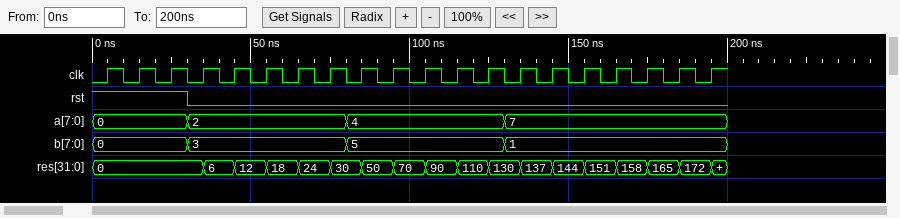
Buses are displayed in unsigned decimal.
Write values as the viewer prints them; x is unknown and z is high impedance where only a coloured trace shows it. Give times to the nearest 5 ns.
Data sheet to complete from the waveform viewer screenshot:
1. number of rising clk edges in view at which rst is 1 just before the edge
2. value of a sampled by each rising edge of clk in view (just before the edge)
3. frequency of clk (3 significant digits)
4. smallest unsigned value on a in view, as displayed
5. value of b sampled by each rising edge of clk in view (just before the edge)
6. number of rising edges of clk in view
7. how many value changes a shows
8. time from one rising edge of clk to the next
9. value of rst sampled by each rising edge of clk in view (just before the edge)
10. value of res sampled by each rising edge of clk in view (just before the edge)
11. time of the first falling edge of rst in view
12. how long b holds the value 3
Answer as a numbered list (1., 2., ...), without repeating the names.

1. 3
2. 0, 0, 0, 2, 2, 2, 2, 2, 4, 4, 4, 4, 4, 7, 7, 7, 7, 7, 7, 7
3. 100 MHz
4. 0
5. 0, 0, 0, 3, 3, 3, 3, 3, 5, 5, 5, 5, 5, 1, 1, 1, 1, 1, 1, 1
6. 20
7. 3
8. 10 ns
9. 1 1 1 0 0 0 0 0 0 0 0 0 0 0 0 0 0 0 0 0
10. 0, 0, 0, 0, 6, 12, 18, 24, 30, 50, 70, 90, 110, 130, 137, 144, 151, 158, 165, 172
11. 30 ns
12. 50 ns
